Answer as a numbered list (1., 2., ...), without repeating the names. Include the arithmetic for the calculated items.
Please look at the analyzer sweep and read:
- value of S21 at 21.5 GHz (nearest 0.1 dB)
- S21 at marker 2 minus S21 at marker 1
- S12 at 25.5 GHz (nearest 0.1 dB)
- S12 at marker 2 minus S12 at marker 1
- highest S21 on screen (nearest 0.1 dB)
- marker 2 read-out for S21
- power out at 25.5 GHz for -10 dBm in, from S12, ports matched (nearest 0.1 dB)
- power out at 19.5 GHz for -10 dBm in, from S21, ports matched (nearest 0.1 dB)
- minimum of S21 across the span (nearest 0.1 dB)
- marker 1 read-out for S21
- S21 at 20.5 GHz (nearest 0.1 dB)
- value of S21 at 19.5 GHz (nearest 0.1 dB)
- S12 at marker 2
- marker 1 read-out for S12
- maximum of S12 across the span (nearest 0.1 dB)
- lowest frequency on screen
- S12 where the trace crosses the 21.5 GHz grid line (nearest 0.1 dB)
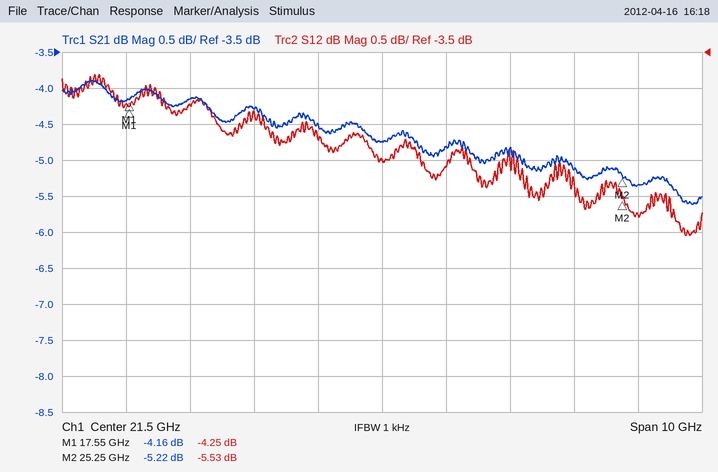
1. -4.7 dB
2. -5.22 − (-4.16) = -1.06 dB
3. -5.8 dB
4. -5.53 − (-4.25) = -1.28 dB
5. -3.9 dB
6. -5.22 dB
7. -10 dBm + (-5.8 dB) = -15.8 dBm
8. -10 dBm + (-4.3 dB) = -14.3 dBm
9. -5.6 dB
10. -4.16 dB
11. -4.5 dB
12. -4.3 dB
13. -5.53 dB
14. -4.25 dB
15. -3.8 dB
16. 16.5 GHz
17. -5.0 dB
